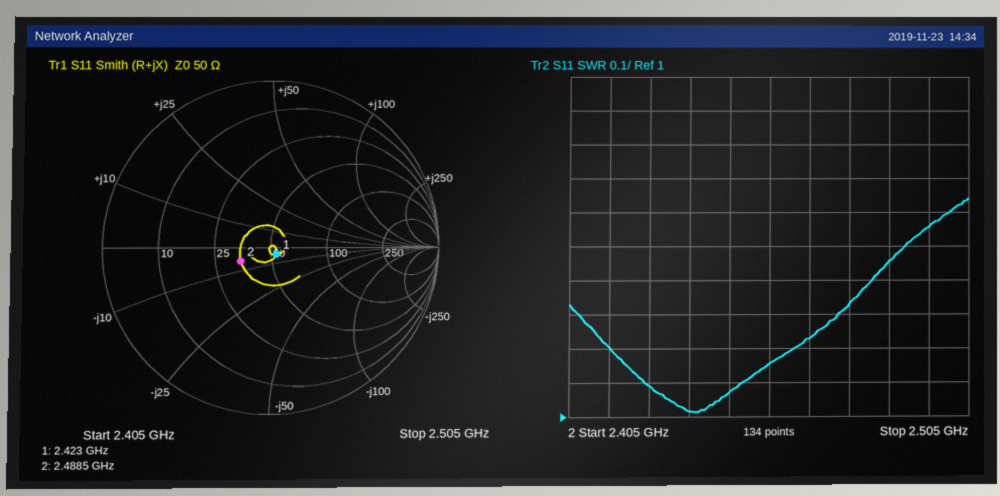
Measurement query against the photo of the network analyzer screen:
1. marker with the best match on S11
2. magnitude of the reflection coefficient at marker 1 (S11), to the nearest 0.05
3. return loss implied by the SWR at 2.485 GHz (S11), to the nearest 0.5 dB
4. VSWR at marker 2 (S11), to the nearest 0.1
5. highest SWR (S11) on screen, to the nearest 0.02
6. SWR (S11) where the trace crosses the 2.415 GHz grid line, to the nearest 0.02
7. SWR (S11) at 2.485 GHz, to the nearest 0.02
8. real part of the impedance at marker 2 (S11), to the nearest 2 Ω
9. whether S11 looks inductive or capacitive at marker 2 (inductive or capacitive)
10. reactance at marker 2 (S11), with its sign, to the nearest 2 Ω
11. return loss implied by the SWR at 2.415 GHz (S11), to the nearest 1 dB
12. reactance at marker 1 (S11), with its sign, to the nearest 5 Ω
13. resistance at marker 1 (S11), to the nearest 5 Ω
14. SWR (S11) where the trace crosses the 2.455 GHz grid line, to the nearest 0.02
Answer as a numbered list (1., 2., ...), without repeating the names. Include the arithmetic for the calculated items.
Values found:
1. marker 1
2. 0.05
3. −20 log10((1.46 − 1)/(1.46 + 1)) ≈ 14.6 dB, so 14.5 dB to the nearest 0.5 dB
4. 1.5
5. 1.64
6. 1.20
7. 1.46
8. 34 Ω
9. capacitive
10. -6 Ω
11. −20 log10((1.2 − 1)/(1.2 + 1)) ≈ 21 dB
12. -5 Ω
13. 55 Ω
14. 1.16
